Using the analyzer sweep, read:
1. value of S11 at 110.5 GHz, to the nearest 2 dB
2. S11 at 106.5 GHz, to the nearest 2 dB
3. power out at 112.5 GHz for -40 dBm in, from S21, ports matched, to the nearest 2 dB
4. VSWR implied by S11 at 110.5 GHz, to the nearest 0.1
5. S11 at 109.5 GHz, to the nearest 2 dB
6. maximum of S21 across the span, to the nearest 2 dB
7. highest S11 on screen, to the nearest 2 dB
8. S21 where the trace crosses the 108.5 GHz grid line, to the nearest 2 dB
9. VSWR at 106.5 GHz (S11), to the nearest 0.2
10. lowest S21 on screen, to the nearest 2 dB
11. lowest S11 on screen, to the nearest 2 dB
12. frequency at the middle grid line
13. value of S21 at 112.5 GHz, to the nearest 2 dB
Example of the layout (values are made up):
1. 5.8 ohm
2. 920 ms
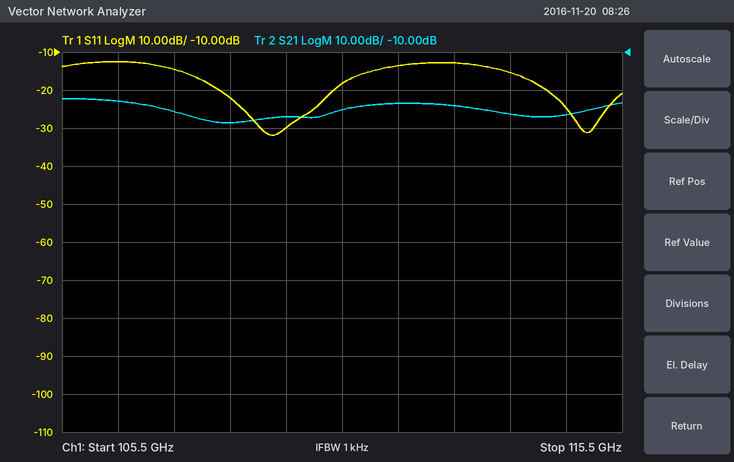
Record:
1. -18 dB
2. -12 dB
3. -64 dBm
4. 1.3
5. -30 dB
6. -22 dB
7. -12 dB
8. -28 dB
9. 1.6
10. -28 dB
11. -32 dB
12. 110.5 GHz
13. -24 dB
